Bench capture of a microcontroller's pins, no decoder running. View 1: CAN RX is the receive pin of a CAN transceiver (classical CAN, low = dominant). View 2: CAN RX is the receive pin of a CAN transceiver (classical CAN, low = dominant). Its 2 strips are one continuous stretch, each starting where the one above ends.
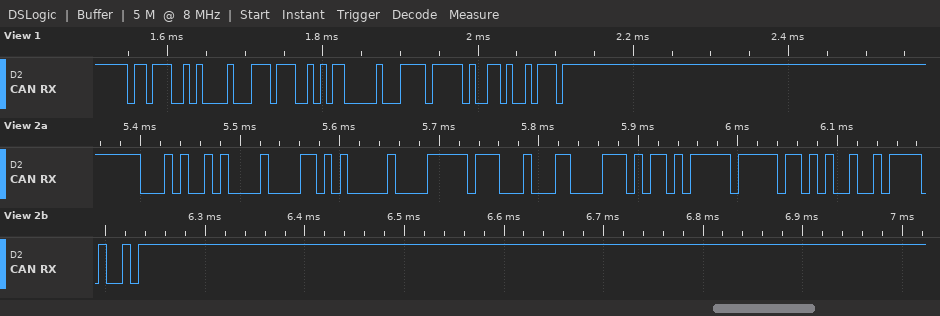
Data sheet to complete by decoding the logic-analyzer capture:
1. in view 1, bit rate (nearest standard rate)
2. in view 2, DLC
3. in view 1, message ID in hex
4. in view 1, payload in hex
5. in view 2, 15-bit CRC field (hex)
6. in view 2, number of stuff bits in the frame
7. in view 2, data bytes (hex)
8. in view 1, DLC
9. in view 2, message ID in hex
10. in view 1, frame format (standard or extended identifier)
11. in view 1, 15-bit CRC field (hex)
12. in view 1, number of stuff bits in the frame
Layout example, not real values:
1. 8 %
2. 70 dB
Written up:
1. 125 kbit/s
2. 8
3. 0x6E5
4. 77 2B 00 F7
5. 0x12F4
6. 4
7. 6A 00 FF 11 87 5A FF F5
8. 4
9. 0x14A
10. standard
11. 0x734B
12. 2
